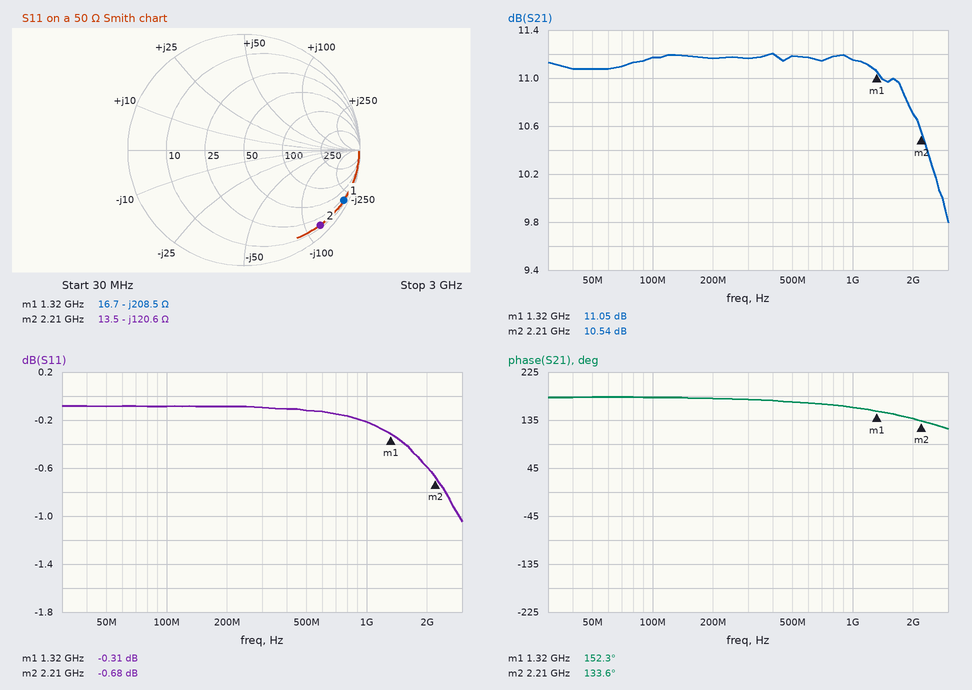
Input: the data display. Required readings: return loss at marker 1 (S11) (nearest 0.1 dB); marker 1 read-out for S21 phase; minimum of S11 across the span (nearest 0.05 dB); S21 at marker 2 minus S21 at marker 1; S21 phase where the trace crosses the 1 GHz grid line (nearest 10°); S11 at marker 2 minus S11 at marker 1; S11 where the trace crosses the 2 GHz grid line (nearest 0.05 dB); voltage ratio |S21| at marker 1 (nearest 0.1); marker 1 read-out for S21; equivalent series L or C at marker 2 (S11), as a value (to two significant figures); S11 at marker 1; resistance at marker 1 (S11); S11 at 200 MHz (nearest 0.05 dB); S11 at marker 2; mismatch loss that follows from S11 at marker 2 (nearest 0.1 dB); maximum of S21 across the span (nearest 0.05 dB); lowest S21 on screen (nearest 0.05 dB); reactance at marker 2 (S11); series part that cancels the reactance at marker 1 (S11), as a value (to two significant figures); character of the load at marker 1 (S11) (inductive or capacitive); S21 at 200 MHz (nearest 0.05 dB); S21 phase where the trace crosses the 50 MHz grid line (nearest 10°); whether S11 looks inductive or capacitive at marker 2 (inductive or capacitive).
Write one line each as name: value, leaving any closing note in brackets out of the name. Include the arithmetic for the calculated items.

return loss at marker 1 (S11): 0.3 dB
marker 1 read-out for S21 phase: 152.3°
minimum of S11 across the span: -1.05 dB
S21 at marker 2 minus S21 at marker 1: 10.54 − (11.05) = -0.51 dB
S21 phase where the trace crosses the 1 GHz grid line: 160°
S11 at marker 2 minus S11 at marker 1: -0.68 − (-0.31) = -0.37 dB
S11 where the trace crosses the 2 GHz grid line: -0.60 dB
voltage ratio |S21| at marker 1: 10^(11.05/20) ≈ 3.6
marker 1 read-out for S21: 11.05 dB
equivalent series L or C at marker 2 (S11), as a value: C = 1/(2π × 2.21 GHz × 120.6 Ω) ≈ 597 fF, so 600 fF to two significant figures
S11 at marker 1: -0.31 dB
resistance at marker 1: 16.7 Ω
S11 at 200 MHz: -0.10 dB
S11 at marker 2: -0.68 dB
mismatch loss that follows from S11 at marker 2: −10 log10(1 − 10^(-0.68/10)) ≈ 8.4 dB
maximum of S21 across the span: 11.20 dB
lowest S21 on screen: 9.80 dB
reactance at marker 2: -120.6 Ω
series part that cancels the reactance at marker 1 (S11), as a value: L = 208.5 Ω/(2π × 1.32 GHz) ≈ 25 nH
character of the load at marker 1 (S11): capacitive
S21 at 200 MHz: 11.15 dB
S21 phase where the trace crosses the 50 MHz grid line: 180°
whether S11 looks inductive or capacitive at marker 2: capacitive
